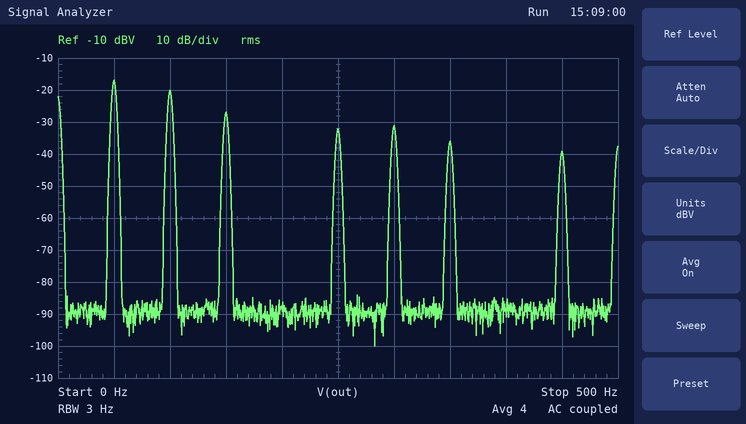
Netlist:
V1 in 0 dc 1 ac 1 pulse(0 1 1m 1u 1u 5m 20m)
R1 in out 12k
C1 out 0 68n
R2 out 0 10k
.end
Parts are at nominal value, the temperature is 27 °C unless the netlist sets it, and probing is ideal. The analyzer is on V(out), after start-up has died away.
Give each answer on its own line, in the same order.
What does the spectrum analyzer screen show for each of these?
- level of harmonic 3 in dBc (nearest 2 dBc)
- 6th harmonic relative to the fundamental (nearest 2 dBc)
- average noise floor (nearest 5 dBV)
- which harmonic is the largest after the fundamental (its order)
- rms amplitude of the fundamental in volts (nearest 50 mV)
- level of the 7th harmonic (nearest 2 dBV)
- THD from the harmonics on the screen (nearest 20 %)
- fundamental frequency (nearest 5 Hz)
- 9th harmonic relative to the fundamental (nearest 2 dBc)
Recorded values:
-10 dBc
-14 dBc
-90 dBV
2
150 mV
-36 dBV
80 %
50 Hz
-22 dBc
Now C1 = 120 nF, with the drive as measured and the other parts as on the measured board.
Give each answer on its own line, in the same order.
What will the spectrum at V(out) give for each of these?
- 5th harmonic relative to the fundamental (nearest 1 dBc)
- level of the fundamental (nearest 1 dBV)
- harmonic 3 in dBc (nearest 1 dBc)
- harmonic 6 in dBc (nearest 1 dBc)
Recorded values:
-17 dBc
-17 dBV
-11 dBc
-16 dBc
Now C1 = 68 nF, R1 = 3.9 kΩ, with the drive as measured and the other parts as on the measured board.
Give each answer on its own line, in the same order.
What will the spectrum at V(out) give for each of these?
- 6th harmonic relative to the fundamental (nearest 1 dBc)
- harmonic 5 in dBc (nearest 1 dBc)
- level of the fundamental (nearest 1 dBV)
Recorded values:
-13 dBc
-14 dBc
-13 dBV
